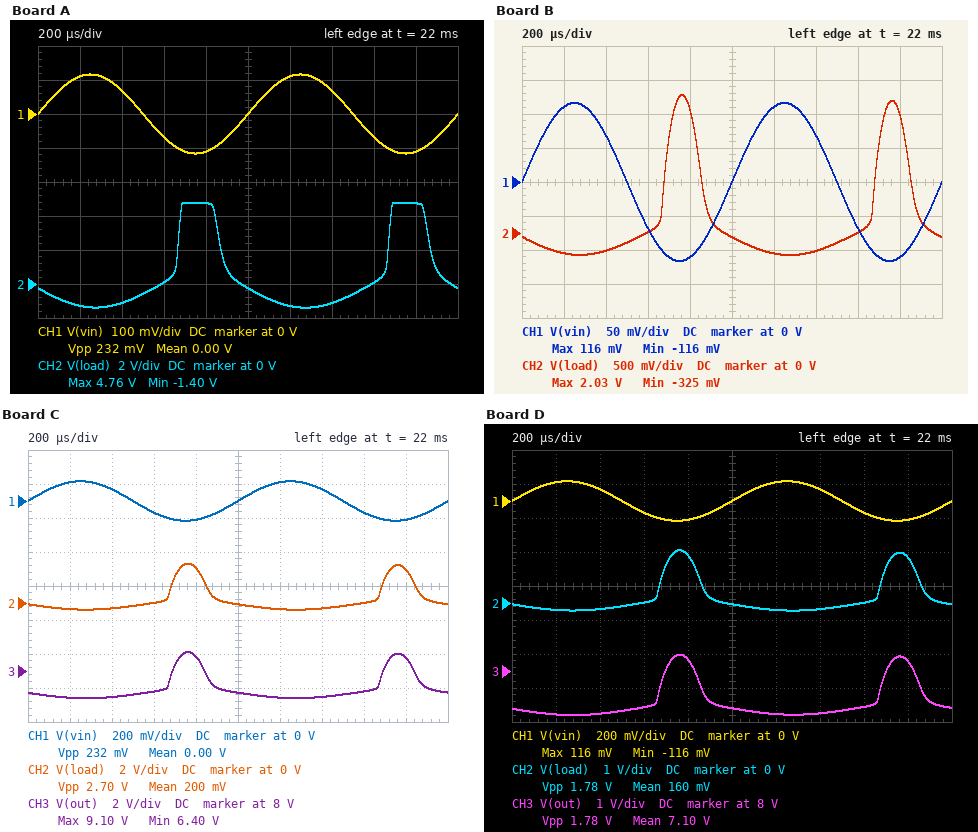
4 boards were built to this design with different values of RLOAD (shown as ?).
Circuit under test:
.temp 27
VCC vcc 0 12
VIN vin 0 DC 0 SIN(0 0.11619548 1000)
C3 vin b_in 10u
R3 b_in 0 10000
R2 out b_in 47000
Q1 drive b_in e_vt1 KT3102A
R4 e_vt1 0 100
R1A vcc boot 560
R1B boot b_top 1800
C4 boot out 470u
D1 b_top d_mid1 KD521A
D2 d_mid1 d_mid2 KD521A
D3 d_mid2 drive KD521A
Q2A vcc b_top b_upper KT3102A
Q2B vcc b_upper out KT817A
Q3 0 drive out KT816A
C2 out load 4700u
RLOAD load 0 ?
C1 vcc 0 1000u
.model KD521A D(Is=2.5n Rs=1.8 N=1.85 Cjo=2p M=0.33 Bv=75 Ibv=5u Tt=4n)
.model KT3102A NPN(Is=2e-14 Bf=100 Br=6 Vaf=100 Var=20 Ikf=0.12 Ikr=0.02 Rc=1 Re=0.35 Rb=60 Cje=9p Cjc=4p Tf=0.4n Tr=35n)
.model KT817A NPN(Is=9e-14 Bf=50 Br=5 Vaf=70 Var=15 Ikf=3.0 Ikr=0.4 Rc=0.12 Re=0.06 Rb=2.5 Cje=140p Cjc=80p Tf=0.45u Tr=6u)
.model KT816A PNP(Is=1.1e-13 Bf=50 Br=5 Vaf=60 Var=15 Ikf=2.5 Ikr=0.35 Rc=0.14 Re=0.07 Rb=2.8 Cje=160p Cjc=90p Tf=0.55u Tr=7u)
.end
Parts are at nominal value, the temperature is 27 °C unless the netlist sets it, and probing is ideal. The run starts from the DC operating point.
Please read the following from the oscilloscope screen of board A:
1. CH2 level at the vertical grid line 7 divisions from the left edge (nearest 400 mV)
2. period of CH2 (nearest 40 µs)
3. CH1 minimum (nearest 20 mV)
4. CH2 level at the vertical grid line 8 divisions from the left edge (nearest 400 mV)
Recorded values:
-1.2 V
1.00 ms
-120 mV
0 V
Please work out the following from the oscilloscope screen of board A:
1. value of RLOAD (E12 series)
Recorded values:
18 Ω
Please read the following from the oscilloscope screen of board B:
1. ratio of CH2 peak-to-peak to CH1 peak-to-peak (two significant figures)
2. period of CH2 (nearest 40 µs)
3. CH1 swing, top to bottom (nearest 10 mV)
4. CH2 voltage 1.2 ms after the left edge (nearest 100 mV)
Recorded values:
10
1.00 ms
230 mV
-300 mV
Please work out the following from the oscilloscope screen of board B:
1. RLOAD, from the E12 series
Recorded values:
3.9 Ω
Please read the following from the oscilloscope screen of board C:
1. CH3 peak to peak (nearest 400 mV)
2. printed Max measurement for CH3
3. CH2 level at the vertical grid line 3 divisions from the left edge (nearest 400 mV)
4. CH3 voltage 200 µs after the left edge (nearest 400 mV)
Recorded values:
2.8 V
9.10 V
0 V
6.4 V
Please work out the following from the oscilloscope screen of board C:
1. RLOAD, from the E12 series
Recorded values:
4.7 Ω
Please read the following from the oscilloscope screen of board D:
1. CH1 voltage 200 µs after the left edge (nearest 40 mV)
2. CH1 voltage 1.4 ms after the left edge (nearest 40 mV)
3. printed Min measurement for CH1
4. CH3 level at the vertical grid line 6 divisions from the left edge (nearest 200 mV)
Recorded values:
120 mV
80 mV
-116 mV
6.8 V
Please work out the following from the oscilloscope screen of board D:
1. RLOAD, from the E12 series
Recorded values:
2.7 Ω
